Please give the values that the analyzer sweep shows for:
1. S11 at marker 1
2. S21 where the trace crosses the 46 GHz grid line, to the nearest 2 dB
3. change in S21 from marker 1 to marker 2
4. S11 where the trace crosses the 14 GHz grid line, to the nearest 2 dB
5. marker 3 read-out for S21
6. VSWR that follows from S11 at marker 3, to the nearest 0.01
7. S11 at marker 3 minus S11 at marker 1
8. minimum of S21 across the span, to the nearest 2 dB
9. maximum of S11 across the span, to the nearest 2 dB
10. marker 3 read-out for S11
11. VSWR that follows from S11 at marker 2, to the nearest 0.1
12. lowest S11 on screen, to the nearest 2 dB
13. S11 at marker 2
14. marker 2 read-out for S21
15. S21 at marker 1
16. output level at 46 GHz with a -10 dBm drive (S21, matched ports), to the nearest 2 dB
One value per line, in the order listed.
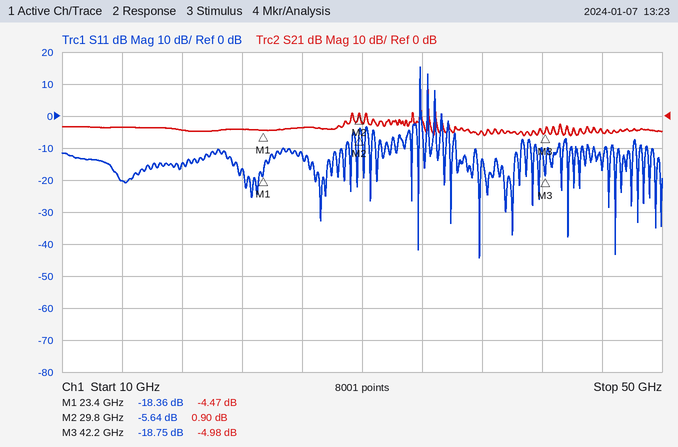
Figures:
-18.36 dB
-4 dB
5.37 dB
-20 dB
-4.98 dB
1.26
-0.39 dB
-6 dB
16 dB
-18.75 dB
3.2
-44 dB
-5.64 dB
0.90 dB
-4.47 dB
-14 dBm
